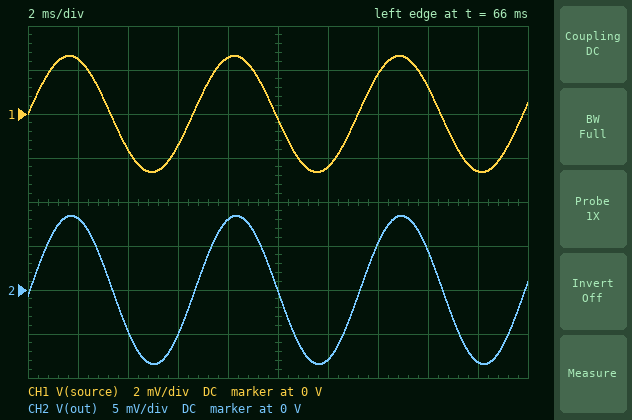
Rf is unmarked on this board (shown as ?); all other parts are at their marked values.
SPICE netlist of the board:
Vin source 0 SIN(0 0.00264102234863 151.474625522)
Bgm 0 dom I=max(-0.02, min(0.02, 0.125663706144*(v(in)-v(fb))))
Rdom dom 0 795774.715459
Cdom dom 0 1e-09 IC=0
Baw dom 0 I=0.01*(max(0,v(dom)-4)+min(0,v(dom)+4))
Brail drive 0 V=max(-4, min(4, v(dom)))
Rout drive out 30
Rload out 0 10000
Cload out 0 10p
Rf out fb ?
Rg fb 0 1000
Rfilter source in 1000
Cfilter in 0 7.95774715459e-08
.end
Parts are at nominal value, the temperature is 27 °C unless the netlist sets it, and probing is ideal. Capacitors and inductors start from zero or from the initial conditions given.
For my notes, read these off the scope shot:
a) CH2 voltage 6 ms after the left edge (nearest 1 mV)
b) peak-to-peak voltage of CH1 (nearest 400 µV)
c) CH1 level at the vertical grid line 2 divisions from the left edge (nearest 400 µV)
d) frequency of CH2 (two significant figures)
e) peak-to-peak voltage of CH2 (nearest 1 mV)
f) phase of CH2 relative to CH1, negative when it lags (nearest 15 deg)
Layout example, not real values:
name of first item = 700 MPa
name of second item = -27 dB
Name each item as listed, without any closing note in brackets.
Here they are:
CH2 voltage 6 ms after the left edge = -5 mV
peak-to-peak voltage of CH1 = 5.2 mV
CH1 level at the vertical grid line 2 divisions from the left edge = -1.6 mV
frequency of CH2 = 150 Hz
peak-to-peak voltage of CH2 = 17 mV
phase of CH2 relative to CH1, negative when it lags = 0 deg
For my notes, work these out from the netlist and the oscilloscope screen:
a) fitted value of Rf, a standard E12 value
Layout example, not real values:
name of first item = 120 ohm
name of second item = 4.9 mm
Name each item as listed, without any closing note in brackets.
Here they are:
fitted value of Rf, a standard E12 value = 2.2 kΩ
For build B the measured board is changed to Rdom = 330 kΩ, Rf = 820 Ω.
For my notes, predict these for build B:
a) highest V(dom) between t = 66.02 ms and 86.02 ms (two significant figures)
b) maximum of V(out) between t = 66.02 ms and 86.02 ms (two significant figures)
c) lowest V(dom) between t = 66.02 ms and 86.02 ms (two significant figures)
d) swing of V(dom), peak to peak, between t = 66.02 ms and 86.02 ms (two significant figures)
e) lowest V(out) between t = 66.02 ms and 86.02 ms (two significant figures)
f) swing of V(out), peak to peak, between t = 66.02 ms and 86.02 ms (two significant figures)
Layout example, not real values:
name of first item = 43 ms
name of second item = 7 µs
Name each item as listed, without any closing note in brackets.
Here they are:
highest V(dom) between t = 66.02 ms and 86.02 ms = 4.9 mV
maximum of V(out) between t = 66.02 ms and 86.02 ms = 4.8 mV
lowest V(dom) between t = 66.02 ms and 86.02 ms = -4.9 mV
swing of V(dom), peak to peak, between t = 66.02 ms and 86.02 ms = 9.8 mV
lowest V(out) between t = 66.02 ms and 86.02 ms = -4.8 mV
swing of V(out), peak to peak, between t = 66.02 ms and 86.02 ms = 9.6 mV
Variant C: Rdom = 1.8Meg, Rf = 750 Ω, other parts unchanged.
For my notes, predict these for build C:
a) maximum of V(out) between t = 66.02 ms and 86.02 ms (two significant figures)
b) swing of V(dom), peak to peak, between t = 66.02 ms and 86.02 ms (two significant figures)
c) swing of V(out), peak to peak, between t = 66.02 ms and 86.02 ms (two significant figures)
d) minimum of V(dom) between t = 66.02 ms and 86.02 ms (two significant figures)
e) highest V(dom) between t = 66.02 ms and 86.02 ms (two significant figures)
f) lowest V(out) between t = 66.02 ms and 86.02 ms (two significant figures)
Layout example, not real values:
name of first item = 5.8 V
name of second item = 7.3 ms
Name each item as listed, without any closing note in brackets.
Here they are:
maximum of V(out) between t = 66.02 ms and 86.02 ms = 4.6 mV
swing of V(dom), peak to peak, between t = 66.02 ms and 86.02 ms = 9.4 mV
swing of V(out), peak to peak, between t = 66.02 ms and 86.02 ms = 9.2 mV
minimum of V(dom) between t = 66.02 ms and 86.02 ms = -4.7 mV
highest V(dom) between t = 66.02 ms and 86.02 ms = 4.7 mV
lowest V(out) between t = 66.02 ms and 86.02 ms = -4.6 mV
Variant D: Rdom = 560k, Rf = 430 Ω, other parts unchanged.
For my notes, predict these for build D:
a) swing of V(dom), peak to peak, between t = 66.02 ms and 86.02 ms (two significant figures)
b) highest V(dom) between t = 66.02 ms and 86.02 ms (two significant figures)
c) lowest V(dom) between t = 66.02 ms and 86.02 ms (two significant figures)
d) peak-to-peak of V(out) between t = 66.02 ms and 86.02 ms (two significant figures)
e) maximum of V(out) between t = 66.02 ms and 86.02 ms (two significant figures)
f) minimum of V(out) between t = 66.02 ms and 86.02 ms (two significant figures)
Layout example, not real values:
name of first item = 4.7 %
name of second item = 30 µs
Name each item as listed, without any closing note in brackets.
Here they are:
swing of V(dom), peak to peak, between t = 66.02 ms and 86.02 ms = 7.7 mV
highest V(dom) between t = 66.02 ms and 86.02 ms = 3.9 mV
lowest V(dom) between t = 66.02 ms and 86.02 ms = -3.9 mV
peak-to-peak of V(out) between t = 66.02 ms and 86.02 ms = 7.5 mV
maximum of V(out) between t = 66.02 ms and 86.02 ms = 3.8 mV
minimum of V(out) between t = 66.02 ms and 86.02 ms = -3.8 mV
